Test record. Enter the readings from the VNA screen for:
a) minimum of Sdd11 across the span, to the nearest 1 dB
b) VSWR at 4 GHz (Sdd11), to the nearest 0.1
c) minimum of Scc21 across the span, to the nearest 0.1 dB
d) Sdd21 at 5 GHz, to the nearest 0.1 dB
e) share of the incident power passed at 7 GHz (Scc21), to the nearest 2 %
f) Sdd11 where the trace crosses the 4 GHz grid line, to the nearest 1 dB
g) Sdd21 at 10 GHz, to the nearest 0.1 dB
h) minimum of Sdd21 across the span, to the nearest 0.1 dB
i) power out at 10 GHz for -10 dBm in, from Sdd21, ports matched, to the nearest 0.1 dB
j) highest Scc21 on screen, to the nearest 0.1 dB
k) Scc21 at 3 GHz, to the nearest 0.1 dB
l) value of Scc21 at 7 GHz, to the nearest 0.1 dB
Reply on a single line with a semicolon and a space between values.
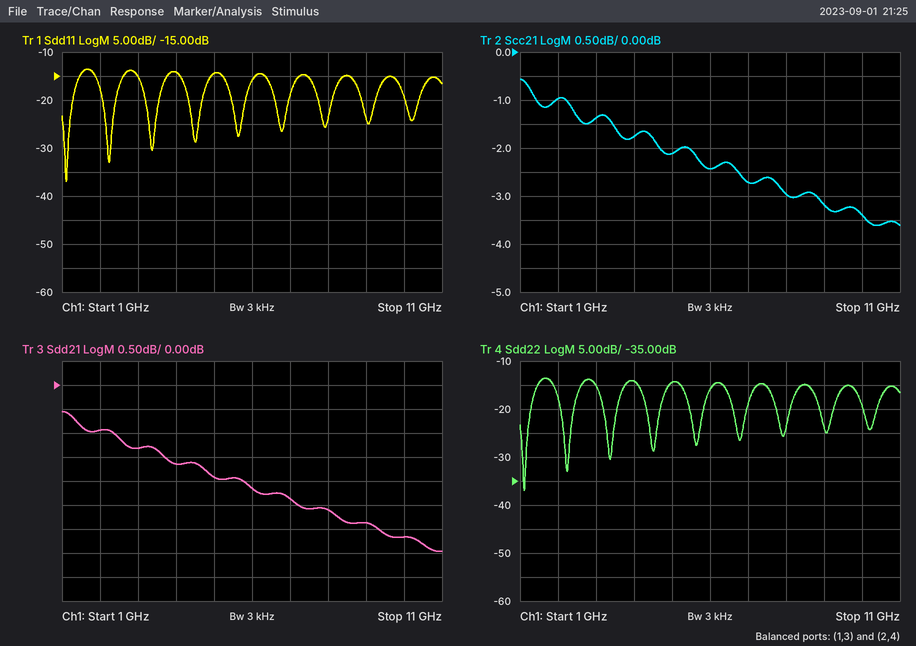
-37 dB; 1.5; -3.6 dB; -1.9 dB; 54 %; -14 dB; -3.2 dB; -3.5 dB; -13.2 dBm; -0.6 dB; -1.4 dB; -2.7 dB
